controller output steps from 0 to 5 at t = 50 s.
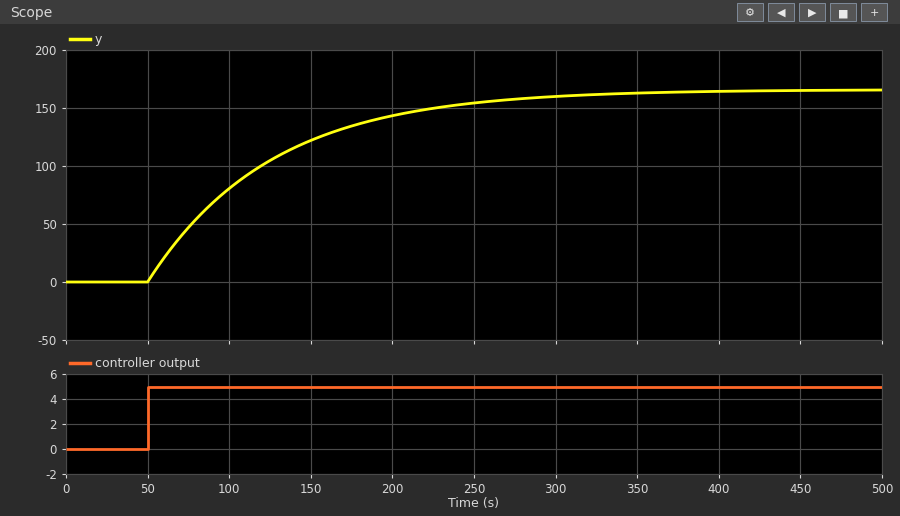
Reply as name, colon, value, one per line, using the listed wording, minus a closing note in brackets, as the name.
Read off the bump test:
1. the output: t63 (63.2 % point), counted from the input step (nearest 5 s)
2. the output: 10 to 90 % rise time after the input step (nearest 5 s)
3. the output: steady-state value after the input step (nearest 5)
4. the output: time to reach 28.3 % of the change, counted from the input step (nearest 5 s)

the output: t63 (63.2 % point), counted from the input step: 75 s
the output: 10 to 90 % rise time after the input step: 165 s
the output: steady-state value after the input step: 165
the output: time to reach 28.3 % of the change, counted from the input step: 25 s
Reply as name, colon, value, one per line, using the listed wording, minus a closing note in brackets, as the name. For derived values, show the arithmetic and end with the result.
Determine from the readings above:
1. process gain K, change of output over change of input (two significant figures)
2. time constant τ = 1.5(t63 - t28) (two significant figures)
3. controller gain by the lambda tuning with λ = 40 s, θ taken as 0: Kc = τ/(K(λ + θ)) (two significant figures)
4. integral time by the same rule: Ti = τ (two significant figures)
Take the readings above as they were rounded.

process gain K, change of output over change of input: (165 - 0) / 5 = 33
time constant τ = 1.5(t63 - t28): 1.5 × (75 - 25) = 75 s
controller gain by the lambda tuning with λ = 40 s, θ taken as 0: Kc = τ/(K(λ + θ)): 75 / (33 × (40 + 0)) = 0.057
integral time by the same rule: Ti = τ: 75 s
